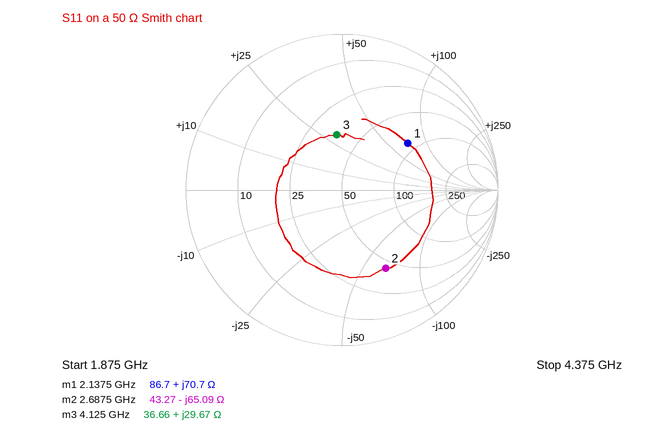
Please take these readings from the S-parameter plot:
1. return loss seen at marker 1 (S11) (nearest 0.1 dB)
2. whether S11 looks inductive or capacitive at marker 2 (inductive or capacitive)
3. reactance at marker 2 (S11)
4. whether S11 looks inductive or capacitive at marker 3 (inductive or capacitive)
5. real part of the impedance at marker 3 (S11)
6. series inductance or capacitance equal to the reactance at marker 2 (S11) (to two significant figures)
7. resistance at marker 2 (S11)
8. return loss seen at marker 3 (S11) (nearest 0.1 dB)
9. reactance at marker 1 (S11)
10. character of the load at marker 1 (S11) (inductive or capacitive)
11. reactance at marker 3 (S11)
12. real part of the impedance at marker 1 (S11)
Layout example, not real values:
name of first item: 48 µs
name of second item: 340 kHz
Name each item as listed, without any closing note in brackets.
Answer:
return loss seen at marker 1 (S11): 5.7 dB
whether S11 looks inductive or capacitive at marker 2: capacitive
reactance at marker 2: -65.09 Ω
whether S11 looks inductive or capacitive at marker 3: inductive
real part of the impedance at marker 3: 36.66 Ω
series inductance or capacitance equal to the reactance at marker 2 (S11): 910 fF
resistance at marker 2: 43.27 Ω
return loss seen at marker 3 (S11): 9.0 dB
reactance at marker 1: +70.7 Ω
character of the load at marker 1 (S11): inductive
reactance at marker 3: +29.67 Ω
real part of the impedance at marker 1: 86.7 Ω
